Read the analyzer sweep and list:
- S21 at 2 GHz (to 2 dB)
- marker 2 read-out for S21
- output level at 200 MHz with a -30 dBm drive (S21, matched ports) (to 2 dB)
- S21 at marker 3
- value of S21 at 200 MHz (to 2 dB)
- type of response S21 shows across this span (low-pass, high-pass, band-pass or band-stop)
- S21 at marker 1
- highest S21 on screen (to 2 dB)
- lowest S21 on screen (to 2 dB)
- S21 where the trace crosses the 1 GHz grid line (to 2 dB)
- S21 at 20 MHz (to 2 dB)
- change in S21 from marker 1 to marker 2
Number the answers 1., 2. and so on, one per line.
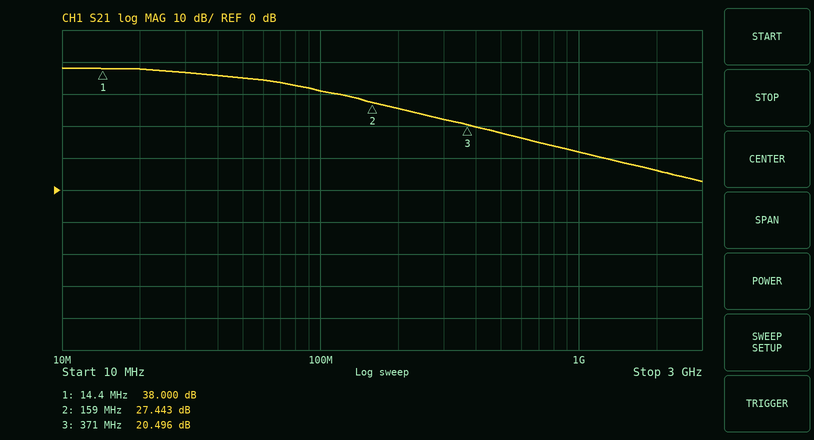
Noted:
1. 6 dB
2. 27.443 dB
3. -4 dBm
4. 20.496 dB
5. 26 dB
6. low-pass
7. 38.000 dB
8. 38 dB
9. 2 dB
10. 12 dB
11. 38 dB
12. -10.557 dB
